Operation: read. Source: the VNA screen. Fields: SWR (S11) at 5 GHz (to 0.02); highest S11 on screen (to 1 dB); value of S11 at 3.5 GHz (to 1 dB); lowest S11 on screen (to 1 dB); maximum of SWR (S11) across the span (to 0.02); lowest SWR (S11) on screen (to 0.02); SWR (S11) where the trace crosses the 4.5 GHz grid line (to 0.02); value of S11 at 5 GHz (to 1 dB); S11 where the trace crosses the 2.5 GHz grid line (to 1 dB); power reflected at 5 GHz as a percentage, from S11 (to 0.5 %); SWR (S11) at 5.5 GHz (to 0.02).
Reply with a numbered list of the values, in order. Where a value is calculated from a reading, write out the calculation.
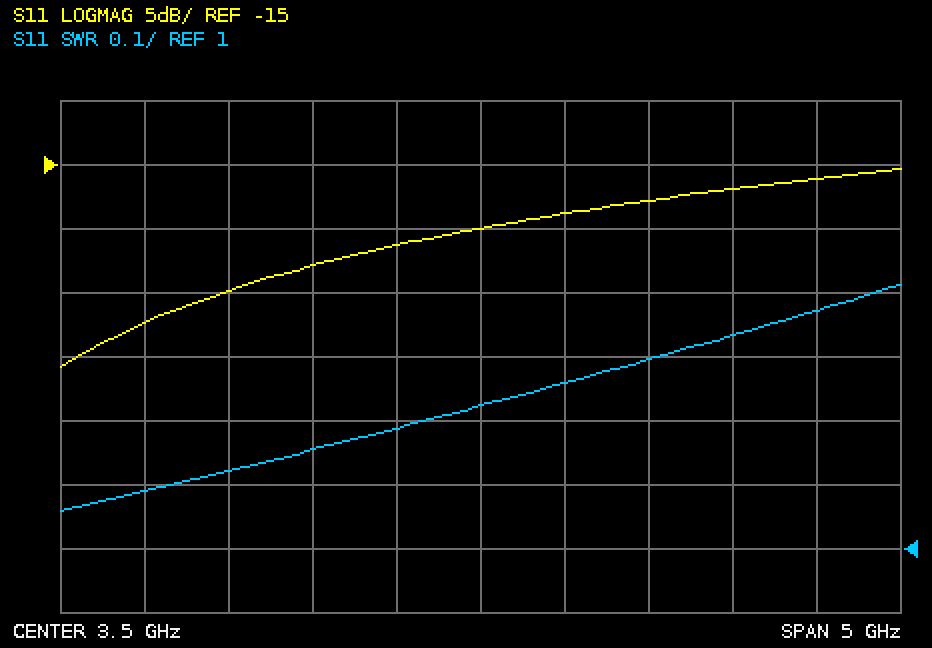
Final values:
1. 1.34
2. -15 dB
3. -20 dB
4. -31 dB
5. 1.42
6. 1.06
7. 1.30
8. -17 dB
9. -23 dB
10. 10^(-17/10) ≈ 2.0 %
11. 1.38
